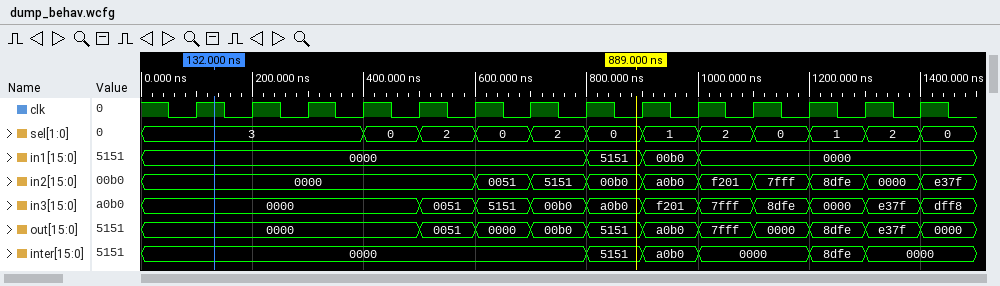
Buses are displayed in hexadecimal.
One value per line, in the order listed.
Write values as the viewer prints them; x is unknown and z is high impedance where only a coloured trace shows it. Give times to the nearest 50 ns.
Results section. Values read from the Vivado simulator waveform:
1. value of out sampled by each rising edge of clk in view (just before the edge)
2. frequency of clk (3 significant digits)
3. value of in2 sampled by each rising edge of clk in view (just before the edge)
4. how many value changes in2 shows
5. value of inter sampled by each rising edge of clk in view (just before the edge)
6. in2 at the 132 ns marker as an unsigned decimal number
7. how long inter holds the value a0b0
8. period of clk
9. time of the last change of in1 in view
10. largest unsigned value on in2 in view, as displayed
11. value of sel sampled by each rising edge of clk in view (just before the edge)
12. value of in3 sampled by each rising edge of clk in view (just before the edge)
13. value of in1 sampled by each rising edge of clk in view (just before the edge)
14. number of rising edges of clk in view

0000, 0000, 0000, 0000, 0000, 0051, 0000, 00b0, 5151, a0b0, 7fff, 0000, 8dfe, e37f
10.0 MHz
0000, 0000, 0000, 0000, 0000, 0000, 0051, 5151, 00b0, a0b0, f201, 7fff, 8dfe, 0000
9
0000, 0000, 0000, 0000, 0000, 0000, 0000, 0000, 5151, a0b0, 0000, 0000, 8dfe, 0000
0
100 ns
100 ns
1000 ns
f201
3, 3, 3, 3, 0, 2, 0, 2, 0, 1, 2, 0, 1, 2
0000, 0000, 0000, 0000, 0000, 0051, 5151, 00b0, a0b0, f201, 7fff, 8dfe, 0000, e37f
0000, 0000, 0000, 0000, 0000, 0000, 0000, 0000, 5151, 00b0, 0000, 0000, 0000, 0000
14
